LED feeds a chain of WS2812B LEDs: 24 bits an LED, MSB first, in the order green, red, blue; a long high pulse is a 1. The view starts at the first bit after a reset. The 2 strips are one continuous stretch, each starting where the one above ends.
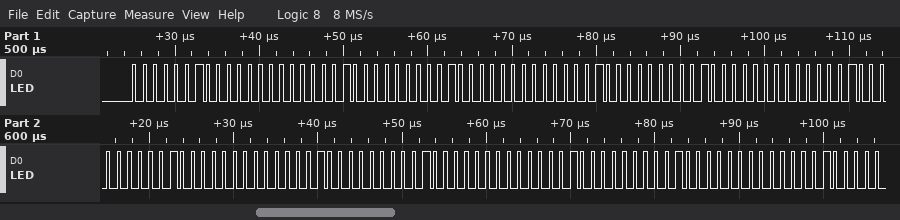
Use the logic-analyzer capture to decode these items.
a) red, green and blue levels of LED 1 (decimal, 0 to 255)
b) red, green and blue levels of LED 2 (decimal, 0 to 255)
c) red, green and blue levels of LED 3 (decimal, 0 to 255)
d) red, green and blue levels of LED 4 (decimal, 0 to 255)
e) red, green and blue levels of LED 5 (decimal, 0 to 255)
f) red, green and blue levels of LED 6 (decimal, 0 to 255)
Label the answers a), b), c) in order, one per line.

a) 0, 2, 8
b) 0, 2, 8
c) 0, 2, 8
d) 0, 2, 8
e) 0, 2, 8
f) 0, 2, 8
